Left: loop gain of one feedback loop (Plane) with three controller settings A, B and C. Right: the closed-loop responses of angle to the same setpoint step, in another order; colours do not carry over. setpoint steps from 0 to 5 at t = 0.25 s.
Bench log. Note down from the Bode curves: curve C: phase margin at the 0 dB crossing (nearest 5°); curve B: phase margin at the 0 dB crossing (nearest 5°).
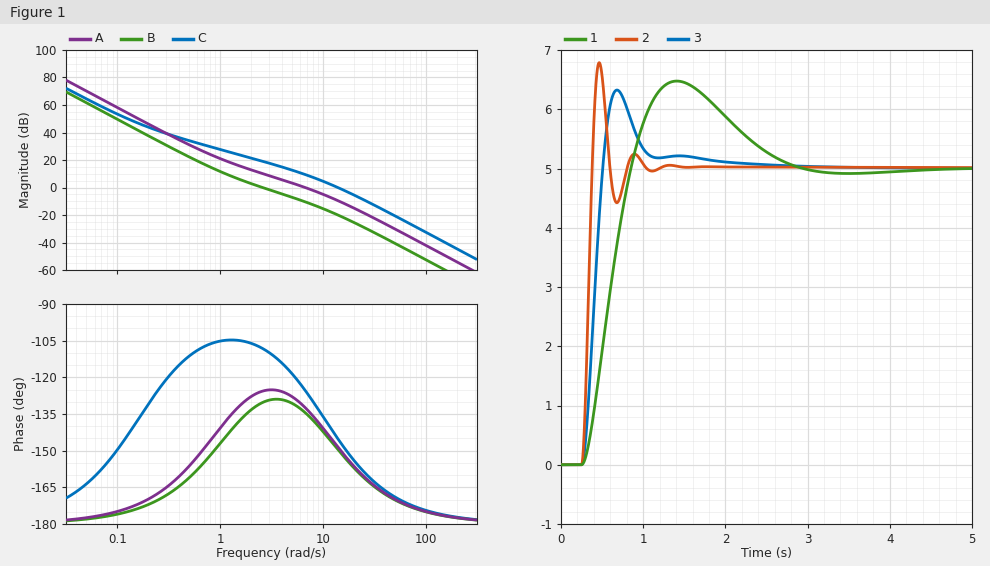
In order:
35°
50°
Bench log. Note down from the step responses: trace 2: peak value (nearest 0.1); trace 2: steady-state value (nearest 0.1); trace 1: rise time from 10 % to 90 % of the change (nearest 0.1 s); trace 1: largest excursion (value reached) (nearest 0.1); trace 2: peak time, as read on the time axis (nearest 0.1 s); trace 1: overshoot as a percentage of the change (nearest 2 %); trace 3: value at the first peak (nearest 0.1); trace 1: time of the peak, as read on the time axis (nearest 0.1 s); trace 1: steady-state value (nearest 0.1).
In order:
6.8
5.0
0.4 s
6.5
0.5 s
30 %
6.3
1.4 s
5.0
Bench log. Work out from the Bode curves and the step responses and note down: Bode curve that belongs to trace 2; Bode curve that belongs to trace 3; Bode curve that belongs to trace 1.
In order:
C
A
B
